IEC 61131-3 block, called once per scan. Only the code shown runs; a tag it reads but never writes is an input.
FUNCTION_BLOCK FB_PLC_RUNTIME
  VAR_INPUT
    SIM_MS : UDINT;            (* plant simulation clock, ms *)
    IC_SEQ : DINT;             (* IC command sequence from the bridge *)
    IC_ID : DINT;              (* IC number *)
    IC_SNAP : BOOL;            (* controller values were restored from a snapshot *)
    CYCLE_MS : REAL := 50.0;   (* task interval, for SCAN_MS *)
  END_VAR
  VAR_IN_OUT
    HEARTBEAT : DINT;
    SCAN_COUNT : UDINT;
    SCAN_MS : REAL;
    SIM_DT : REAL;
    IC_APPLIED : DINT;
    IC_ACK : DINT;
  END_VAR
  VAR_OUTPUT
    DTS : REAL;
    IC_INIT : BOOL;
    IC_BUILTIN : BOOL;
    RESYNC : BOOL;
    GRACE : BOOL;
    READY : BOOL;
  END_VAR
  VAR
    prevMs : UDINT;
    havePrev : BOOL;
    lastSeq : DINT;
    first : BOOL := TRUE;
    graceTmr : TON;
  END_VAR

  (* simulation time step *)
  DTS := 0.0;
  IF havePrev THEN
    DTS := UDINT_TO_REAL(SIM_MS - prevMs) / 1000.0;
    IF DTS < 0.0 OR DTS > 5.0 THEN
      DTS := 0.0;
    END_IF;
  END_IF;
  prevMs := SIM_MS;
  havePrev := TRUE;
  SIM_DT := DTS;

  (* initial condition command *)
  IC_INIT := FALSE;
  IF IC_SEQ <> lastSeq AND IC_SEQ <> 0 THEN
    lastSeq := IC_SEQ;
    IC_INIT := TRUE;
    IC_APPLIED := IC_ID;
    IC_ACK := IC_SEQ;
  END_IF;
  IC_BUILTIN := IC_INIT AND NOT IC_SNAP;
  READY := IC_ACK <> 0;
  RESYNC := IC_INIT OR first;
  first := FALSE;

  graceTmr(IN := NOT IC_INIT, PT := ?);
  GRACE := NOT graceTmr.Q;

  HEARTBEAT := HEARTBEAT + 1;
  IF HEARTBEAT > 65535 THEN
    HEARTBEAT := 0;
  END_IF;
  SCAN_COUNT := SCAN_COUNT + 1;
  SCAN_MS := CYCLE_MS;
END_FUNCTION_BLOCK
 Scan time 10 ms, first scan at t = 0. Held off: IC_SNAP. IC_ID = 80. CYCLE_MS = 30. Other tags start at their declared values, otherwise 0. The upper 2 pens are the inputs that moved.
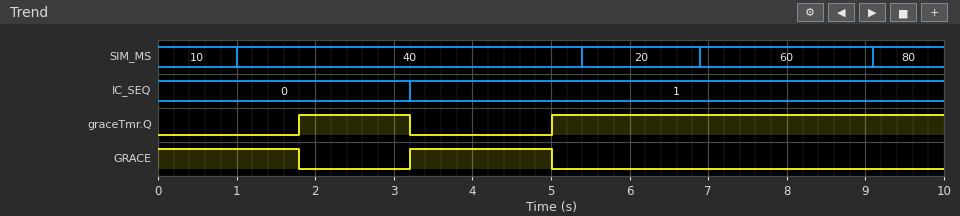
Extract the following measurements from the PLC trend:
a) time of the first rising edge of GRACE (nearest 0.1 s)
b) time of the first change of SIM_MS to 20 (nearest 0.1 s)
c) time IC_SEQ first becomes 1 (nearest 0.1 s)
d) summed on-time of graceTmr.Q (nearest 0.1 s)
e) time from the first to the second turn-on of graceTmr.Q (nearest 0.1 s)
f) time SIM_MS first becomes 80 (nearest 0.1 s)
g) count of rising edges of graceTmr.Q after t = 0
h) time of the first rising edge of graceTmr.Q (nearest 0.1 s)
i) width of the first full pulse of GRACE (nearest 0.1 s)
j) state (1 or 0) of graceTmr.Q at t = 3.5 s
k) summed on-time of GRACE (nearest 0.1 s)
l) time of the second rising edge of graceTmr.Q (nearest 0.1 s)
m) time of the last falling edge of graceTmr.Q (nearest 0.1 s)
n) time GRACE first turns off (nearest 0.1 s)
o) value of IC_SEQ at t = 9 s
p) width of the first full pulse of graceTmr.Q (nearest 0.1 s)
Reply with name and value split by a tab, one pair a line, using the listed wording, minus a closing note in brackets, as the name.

time of the first rising edge of GRACE	3.2 s
time of the first change of SIM_MS to 20	5.4 s
time IC_SEQ first becomes 1	3.2 s
summed on-time of graceTmr.Q	6.4 s
time from the first to the second turn-on of graceTmr.Q	3.2 s
time SIM_MS first becomes 80	9.1 s
count of rising edges of graceTmr.Q after t = 0	2
time of the first rising edge of graceTmr.Q	1.8 s
width of the first full pulse of GRACE	1.8 s
state (1 or 0) of graceTmr.Q at t = 3.5 s	0
summed on-time of GRACE	3.6 s
time of the second rising edge of graceTmr.Q	5.0 s
time of the last falling edge of graceTmr.Q	3.2 s
time GRACE first turns off	1.8 s
value of IC_SEQ at t = 9 s	1
width of the first full pulse of graceTmr.Q	1.4 s
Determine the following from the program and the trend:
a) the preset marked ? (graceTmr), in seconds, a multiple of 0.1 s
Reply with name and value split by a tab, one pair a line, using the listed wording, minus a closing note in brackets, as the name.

the preset marked ? (graceTmr), in seconds, a multiple of 0.1 s	1.8 s
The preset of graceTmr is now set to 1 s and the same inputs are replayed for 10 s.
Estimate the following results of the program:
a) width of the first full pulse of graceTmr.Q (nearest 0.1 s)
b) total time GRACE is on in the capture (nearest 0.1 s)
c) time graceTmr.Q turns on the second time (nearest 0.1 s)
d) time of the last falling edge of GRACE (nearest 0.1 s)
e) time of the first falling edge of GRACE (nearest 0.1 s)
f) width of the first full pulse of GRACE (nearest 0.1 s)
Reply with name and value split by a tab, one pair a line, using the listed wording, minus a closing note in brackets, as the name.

width of the first full pulse of graceTmr.Q	2.2 s
total time GRACE is on in the capture	2.0 s
time graceTmr.Q turns on the second time	4.2 s
time of the last falling edge of GRACE	4.2 s
time of the first falling edge of GRACE	1.0 s
width of the first full pulse of GRACE	1.0 s
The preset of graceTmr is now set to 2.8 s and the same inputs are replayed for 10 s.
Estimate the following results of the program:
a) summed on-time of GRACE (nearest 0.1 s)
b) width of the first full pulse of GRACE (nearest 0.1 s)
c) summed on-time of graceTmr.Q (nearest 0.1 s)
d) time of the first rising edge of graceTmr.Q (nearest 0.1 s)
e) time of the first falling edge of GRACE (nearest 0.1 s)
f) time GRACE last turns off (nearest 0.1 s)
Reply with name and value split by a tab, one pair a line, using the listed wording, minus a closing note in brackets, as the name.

summed on-time of GRACE	5.6 s
width of the first full pulse of GRACE	2.8 s
summed on-time of graceTmr.Q	4.4 s
time of the first rising edge of graceTmr.Q	2.8 s
time of the first falling edge of GRACE	2.8 s
time GRACE last turns off	6.0 s
